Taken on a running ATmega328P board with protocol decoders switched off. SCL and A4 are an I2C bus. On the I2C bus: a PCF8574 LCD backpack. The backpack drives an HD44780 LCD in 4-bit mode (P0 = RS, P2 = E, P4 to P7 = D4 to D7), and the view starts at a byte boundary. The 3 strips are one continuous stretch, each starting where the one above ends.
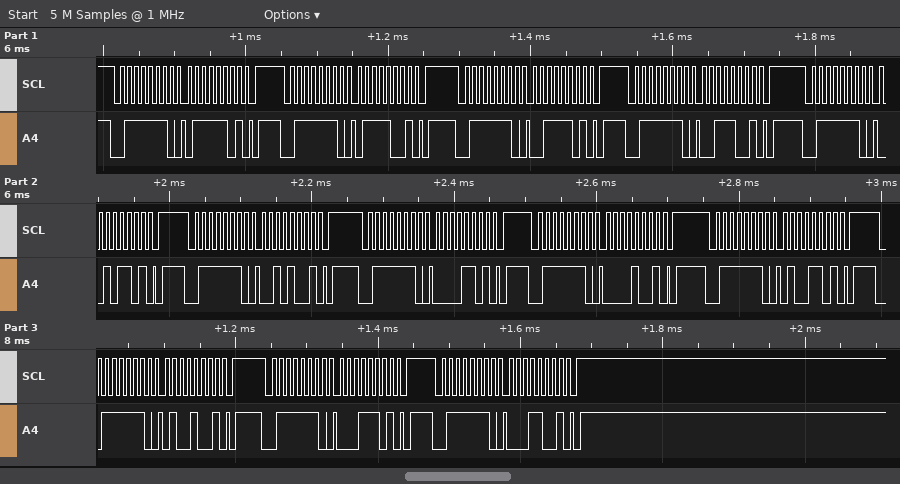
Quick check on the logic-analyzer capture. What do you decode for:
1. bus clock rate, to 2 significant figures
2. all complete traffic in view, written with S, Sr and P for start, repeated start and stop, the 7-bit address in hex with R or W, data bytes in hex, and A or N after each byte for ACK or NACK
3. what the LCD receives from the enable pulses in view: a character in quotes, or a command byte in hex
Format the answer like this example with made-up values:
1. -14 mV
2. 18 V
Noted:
1. 100 kHz
2. S 3FW A 7D A P S 3FW A 79 A P S 3FW A 3D A P S 3FW A 39 A P S 3FW A 2D A P S 3FW A 29 A P S 3FW A 0D A P S 3FW A 09 A P S 3FW A 4D A P S 3FW A 49 A P S 3FW A 1D A P S 3FW A 19 A P
3. 's' ' ' 'A'
